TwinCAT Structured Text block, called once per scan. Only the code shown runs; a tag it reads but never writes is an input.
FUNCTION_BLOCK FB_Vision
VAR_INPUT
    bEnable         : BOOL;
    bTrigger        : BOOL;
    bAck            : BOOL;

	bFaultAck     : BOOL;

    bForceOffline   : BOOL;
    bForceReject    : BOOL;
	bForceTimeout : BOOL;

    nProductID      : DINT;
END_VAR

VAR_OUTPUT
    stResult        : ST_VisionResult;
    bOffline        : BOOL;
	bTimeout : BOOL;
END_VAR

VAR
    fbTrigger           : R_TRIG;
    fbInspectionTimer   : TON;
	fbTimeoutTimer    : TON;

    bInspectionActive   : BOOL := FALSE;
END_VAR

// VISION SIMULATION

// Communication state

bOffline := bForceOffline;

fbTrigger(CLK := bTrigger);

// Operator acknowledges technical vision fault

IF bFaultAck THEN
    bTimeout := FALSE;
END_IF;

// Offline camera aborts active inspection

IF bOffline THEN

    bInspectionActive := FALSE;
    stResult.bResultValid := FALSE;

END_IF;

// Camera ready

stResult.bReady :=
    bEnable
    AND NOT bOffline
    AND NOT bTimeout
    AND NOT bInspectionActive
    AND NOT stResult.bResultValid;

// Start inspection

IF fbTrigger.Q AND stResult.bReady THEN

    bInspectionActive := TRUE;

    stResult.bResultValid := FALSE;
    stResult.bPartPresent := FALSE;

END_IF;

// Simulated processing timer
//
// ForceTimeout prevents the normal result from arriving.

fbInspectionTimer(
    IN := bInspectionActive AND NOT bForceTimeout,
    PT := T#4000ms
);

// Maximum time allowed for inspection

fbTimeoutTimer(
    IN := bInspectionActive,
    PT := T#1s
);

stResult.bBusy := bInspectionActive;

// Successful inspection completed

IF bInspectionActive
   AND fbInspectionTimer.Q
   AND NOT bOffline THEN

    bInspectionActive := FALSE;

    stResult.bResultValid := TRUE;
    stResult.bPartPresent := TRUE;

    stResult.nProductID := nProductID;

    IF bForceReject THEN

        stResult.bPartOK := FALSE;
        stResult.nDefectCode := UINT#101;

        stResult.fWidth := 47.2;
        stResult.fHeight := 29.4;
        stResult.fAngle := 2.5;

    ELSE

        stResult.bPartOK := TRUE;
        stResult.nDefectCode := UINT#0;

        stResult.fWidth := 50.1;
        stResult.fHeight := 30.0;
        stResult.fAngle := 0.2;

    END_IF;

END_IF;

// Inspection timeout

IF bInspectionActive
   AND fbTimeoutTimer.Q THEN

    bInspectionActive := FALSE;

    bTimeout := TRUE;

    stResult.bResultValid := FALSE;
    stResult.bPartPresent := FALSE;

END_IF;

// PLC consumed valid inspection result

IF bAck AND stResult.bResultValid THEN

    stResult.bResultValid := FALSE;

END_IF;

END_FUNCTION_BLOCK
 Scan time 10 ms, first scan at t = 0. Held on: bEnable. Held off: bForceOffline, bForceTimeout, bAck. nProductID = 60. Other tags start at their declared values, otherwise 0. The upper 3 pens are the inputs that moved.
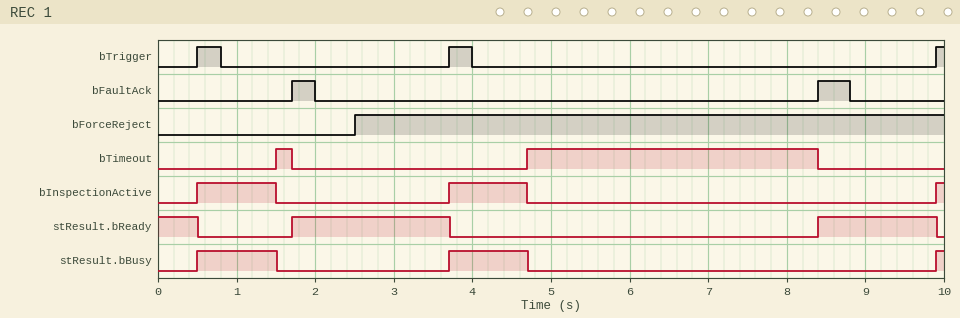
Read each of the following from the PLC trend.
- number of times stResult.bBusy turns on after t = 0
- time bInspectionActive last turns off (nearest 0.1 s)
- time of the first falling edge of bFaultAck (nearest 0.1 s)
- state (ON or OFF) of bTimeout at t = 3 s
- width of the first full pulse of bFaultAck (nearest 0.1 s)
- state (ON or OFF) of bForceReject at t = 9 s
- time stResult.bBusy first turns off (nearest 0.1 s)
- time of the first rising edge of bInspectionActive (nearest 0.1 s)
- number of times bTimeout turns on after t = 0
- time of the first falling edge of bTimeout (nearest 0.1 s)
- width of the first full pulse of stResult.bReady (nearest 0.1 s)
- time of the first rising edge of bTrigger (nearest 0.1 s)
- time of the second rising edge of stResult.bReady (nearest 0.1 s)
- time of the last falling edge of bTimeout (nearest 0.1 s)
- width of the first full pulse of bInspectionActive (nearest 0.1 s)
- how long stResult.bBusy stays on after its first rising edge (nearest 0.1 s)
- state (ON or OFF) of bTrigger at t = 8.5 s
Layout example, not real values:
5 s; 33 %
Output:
3; 4.7 s; 2.0 s; OFF; 0.3 s; ON; 1.5 s; 0.5 s; 2; 1.7 s; 2.0 s; 0.5 s; 8.4 s; 8.4 s; 1.0 s; 1.0 s; OFF
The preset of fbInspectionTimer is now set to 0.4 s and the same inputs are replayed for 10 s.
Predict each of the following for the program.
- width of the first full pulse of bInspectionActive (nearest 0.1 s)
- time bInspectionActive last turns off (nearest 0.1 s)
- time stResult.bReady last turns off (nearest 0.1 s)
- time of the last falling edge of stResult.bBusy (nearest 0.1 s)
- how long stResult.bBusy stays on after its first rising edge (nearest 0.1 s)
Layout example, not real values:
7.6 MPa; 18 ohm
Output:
0.4 s; 0.9 s; 0.5 s; 0.9 s; 0.4 s
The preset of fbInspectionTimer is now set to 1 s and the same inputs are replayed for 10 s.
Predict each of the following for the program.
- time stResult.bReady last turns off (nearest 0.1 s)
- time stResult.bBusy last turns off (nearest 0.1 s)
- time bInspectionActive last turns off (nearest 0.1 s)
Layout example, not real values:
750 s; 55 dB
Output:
0.5 s; 1.5 s; 1.5 s
